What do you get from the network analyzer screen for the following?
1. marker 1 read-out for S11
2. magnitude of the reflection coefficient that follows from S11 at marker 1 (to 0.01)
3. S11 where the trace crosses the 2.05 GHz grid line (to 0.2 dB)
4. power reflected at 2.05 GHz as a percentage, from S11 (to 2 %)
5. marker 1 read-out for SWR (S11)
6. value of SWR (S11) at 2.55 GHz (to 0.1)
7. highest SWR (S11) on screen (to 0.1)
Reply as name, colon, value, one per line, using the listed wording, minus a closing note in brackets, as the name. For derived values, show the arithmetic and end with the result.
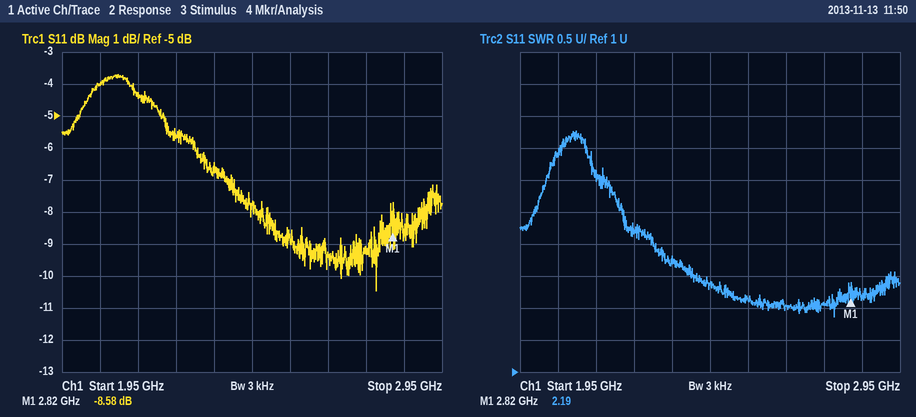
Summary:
marker 1 read-out for S11: -8.58 dB
magnitude of the reflection coefficient that follows from S11 at marker 1: 10^(-8.58/20) ≈ 0.37
S11 where the trace crosses the 2.05 GHz grid line: -4.0 dB
power reflected at 2.05 GHz as a percentage, from S11: 10^(-4/10) ≈ 40 %
marker 1 read-out for SWR: 2.19
value of SWR (S11) at 2.55 GHz: 2.1
highest SWR (S11) on screen: 4.8
